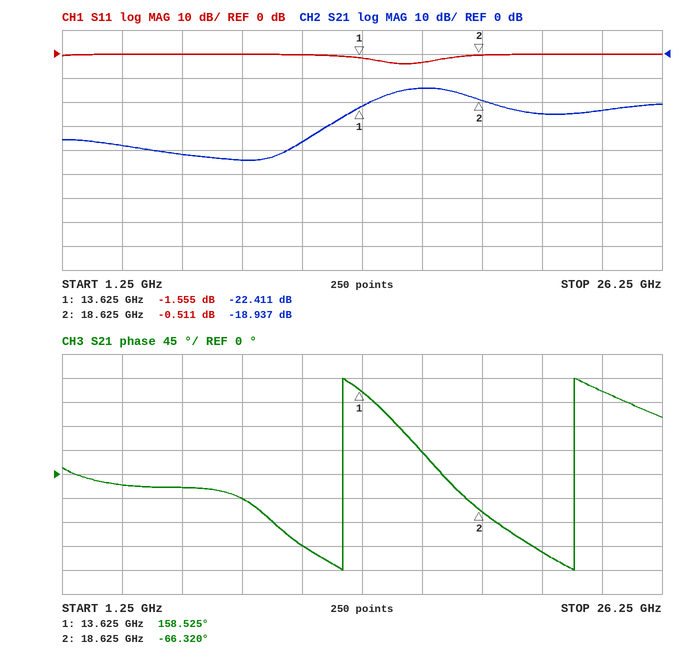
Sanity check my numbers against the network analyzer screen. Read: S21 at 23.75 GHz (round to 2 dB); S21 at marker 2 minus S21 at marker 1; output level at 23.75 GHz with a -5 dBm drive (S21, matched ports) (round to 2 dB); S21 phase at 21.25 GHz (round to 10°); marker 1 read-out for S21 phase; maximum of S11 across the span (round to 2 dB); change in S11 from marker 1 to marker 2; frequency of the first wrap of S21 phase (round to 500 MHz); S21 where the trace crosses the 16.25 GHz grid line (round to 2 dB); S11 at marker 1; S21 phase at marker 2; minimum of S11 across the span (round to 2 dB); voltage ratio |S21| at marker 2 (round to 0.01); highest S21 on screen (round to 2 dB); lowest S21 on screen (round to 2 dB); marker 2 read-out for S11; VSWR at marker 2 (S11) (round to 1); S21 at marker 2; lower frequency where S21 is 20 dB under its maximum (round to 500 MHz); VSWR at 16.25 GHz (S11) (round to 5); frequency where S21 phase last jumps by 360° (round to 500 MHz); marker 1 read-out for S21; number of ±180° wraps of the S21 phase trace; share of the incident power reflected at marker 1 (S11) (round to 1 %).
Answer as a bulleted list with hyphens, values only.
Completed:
- -24 dB
- 3.474 dB
- -28 dBm
- -150°
- 158.525°
- 0 dB
- 1.044 dB
- 13.0 GHz
- -14 dB
- -1.555 dB
- -66.320°
- -4 dB
- 0.11
- -14 dB
- -44 dB
- -0.511 dB
- 34
- -18.937 dB
- 11.5 GHz
- 5
- 22.5 GHz
- -22.411 dB
- 2
- 70 %
